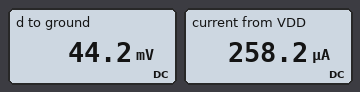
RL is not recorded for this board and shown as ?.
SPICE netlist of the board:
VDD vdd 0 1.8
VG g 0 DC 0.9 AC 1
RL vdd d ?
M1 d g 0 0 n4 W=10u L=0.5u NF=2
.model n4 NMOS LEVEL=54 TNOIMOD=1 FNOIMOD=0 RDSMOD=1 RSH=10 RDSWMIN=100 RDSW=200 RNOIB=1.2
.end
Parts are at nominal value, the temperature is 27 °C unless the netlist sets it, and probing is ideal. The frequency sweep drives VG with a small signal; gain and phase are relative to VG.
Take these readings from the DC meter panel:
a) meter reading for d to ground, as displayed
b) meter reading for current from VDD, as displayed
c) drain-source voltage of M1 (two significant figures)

44.2 mV
258.2 µA
44 mV
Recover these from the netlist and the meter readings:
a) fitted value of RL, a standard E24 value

6.8 kΩ
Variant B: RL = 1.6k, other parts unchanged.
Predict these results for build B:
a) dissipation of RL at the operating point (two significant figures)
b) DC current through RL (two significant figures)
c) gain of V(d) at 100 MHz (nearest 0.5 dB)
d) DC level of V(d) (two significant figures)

1.6 mW
990 µA
-8.0 dB
210 mV
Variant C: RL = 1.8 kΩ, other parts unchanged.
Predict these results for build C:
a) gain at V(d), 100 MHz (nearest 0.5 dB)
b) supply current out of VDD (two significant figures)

-9.5 dB
900 µA
